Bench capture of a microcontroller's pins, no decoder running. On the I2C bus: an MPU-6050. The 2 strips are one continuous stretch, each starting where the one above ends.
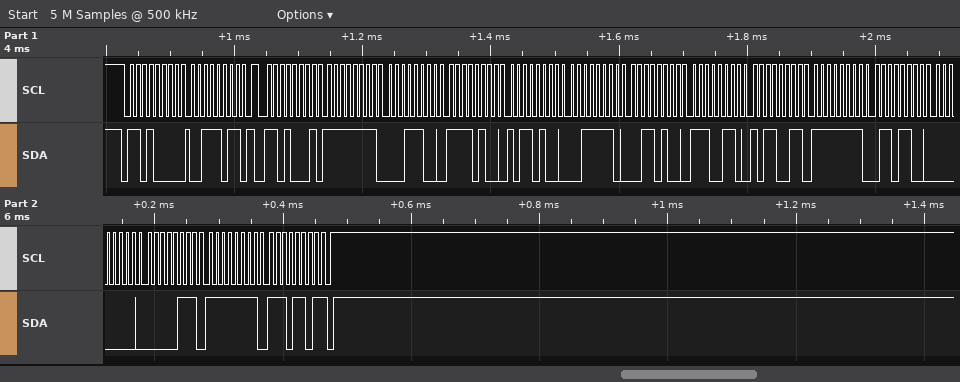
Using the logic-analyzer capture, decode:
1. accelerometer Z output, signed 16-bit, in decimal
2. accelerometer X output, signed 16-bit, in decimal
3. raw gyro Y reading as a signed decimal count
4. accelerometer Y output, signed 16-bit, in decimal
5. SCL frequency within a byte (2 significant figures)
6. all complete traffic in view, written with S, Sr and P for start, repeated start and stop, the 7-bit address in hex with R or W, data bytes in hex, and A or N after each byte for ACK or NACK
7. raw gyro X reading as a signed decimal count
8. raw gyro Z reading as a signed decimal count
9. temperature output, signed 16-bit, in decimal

15924
-228
7
-2892
100 kHz
S 68W A 3B A Sr 68R A FF A 1C A F4 A B4 A 3E A 34 A E6 A B3 A FF A 6C A 00 A 07 A FF A ED N P
-148
-19
-6477
